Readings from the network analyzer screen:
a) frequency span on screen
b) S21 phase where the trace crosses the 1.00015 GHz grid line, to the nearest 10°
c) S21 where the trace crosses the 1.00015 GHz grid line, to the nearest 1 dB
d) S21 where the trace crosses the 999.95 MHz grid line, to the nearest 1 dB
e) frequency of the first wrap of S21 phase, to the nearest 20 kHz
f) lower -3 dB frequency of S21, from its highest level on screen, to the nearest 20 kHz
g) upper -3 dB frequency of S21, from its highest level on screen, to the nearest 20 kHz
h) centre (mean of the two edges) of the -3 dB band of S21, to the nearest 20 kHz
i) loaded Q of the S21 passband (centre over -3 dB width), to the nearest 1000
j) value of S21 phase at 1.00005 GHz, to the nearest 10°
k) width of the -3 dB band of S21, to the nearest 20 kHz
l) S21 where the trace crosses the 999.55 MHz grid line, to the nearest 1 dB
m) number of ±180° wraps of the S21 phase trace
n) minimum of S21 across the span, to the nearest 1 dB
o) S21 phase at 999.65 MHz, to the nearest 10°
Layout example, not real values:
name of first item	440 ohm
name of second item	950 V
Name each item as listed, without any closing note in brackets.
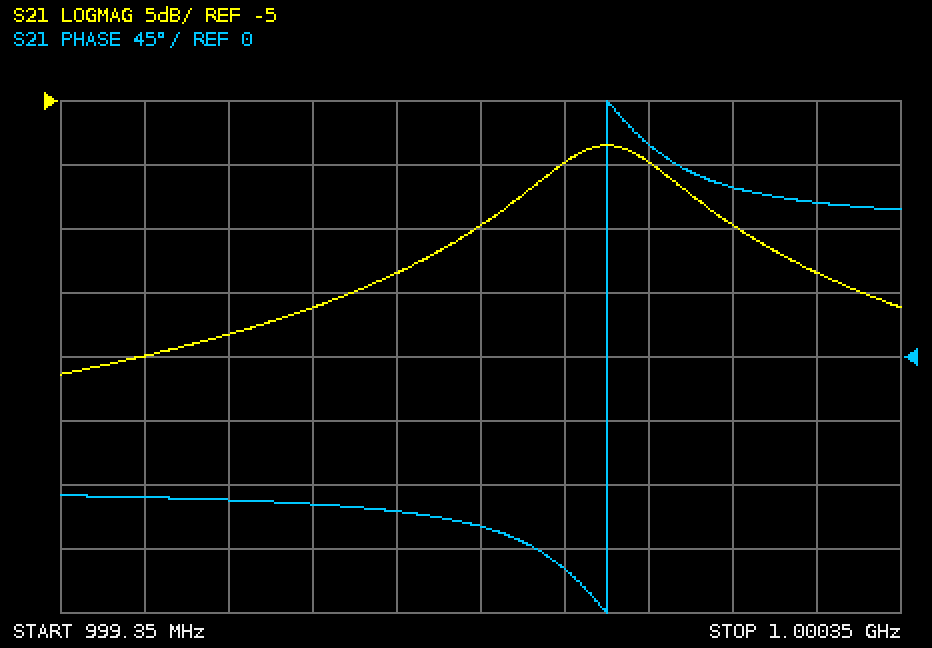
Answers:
frequency span on screen	1 MHz
S21 phase where the trace crosses the 1.00015 GHz grid line, to the nearest 10°	120°
S21 where the trace crosses the 1.00015 GHz grid line, to the nearest 1 dB	-15 dB
S21 where the trace crosses the 999.95 MHz grid line, to the nearest 1 dB	-10 dB
frequency of the first wrap of S21 phase, to the nearest 20 kHz	1.00000 GHz
lower -3 dB frequency of S21, from its highest level on screen, to the nearest 20 kHz	999.92 MHz
upper -3 dB frequency of S21, from its highest level on screen, to the nearest 20 kHz	1.00008 GHz
centre (mean of the two edges) of the -3 dB band of S21, to the nearest 20 kHz	1.00000 GHz
loaded Q of the S21 passband (centre over -3 dB width), to the nearest 1000	6000
value of S21 phase at 1.00005 GHz, to the nearest 10°	150°
width of the -3 dB band of S21, to the nearest 20 kHz	160 kHz
S21 where the trace crosses the 999.55 MHz grid line, to the nearest 1 dB	-23 dB
number of ±180° wraps of the S21 phase trace	1
minimum of S21 across the span, to the nearest 1 dB	-26 dB
S21 phase at 999.65 MHz, to the nearest 10°	-100°
